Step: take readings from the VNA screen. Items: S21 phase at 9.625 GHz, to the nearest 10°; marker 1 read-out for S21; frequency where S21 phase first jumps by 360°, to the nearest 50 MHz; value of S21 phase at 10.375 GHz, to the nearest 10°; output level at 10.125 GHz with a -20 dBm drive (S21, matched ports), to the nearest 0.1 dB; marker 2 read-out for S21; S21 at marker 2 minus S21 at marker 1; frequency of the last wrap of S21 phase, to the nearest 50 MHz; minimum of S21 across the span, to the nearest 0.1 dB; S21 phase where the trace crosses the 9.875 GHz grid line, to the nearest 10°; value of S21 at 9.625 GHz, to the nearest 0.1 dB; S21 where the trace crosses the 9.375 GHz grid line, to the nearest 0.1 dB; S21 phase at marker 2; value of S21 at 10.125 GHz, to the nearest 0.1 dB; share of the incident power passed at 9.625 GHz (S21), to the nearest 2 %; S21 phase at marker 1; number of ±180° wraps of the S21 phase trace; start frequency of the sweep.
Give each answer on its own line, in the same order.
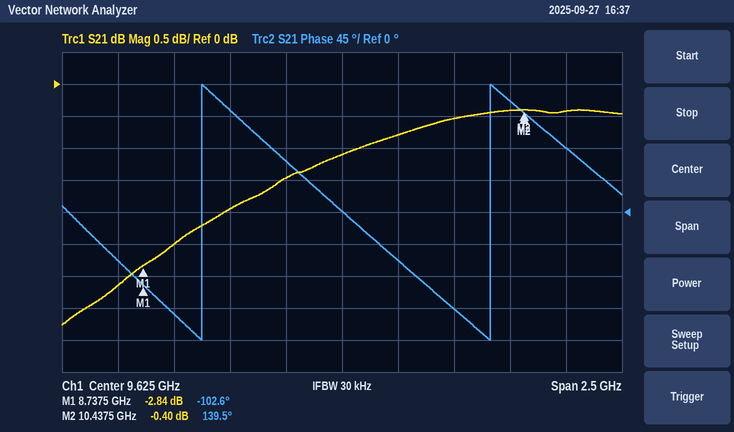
0°
-2.84 dB
9.00 GHz
160°
-20.5 dBm
-0.40 dB
2.44 dB
10.30 GHz
-3.8 dB
-70°
-1.1 dB
-1.5 dB
139.5°
-0.5 dB
78 %
-102.6°
2
8.375 GHz
